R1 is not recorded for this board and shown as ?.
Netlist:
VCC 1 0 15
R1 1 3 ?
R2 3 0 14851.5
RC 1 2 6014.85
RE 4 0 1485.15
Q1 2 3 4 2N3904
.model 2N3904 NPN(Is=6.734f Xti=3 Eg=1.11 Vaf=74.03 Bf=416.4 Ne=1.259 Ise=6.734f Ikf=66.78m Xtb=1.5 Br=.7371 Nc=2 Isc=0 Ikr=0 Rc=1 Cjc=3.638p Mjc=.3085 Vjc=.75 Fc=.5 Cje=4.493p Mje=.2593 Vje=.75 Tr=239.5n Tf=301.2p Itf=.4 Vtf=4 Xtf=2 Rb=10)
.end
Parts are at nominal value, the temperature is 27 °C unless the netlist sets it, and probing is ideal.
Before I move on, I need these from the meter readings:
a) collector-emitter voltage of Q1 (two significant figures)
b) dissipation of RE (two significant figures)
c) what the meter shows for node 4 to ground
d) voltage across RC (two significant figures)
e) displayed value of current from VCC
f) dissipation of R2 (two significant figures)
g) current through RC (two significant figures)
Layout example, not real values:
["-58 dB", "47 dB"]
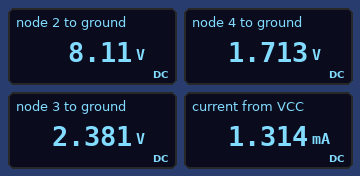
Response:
["6.4 V", "2.0 mW", "1.713 V", "6.9 V", "1.314 mA", "380 µW", "1.1 mA"]
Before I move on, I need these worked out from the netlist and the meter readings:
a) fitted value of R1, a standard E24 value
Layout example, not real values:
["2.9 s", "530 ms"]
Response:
["75 kΩ"]
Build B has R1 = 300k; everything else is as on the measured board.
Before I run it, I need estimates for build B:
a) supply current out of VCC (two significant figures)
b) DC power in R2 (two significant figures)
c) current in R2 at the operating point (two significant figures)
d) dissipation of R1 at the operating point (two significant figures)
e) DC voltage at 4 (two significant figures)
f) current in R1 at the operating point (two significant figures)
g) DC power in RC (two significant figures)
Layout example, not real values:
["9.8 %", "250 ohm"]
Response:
["120 µA", "33 µW", "47 µA", "680 µW", "110 mV", "48 µA", "30 µW"]
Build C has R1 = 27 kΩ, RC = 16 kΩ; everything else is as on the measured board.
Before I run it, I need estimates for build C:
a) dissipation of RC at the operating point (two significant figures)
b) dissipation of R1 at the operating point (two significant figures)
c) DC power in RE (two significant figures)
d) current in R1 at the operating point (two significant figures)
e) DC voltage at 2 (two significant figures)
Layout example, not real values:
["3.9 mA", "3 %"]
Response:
["11 mW", "5.9 mW", "1.9 mW", "470 µA", "1.7 V"]
